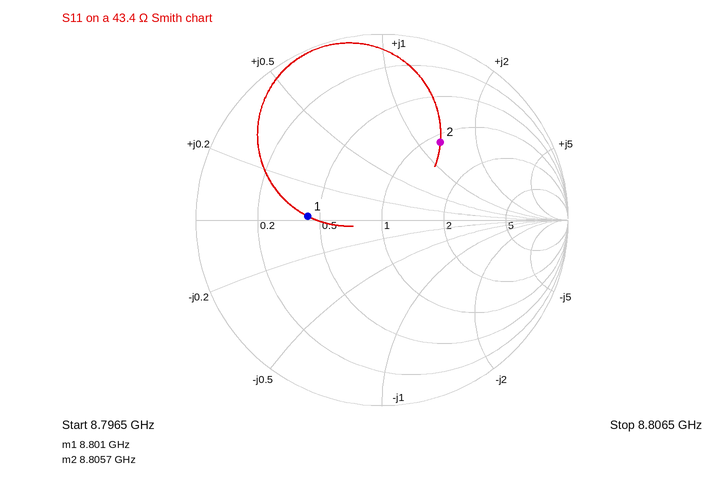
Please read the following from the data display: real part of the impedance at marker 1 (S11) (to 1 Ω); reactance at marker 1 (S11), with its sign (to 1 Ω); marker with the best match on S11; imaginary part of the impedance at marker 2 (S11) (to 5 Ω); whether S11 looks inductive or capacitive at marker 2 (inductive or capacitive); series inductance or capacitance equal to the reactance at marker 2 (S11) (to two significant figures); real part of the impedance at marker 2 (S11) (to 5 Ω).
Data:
19 Ω
+1 Ω
marker 1
+55 Ω
inductive
1.0 nH
50 Ω
